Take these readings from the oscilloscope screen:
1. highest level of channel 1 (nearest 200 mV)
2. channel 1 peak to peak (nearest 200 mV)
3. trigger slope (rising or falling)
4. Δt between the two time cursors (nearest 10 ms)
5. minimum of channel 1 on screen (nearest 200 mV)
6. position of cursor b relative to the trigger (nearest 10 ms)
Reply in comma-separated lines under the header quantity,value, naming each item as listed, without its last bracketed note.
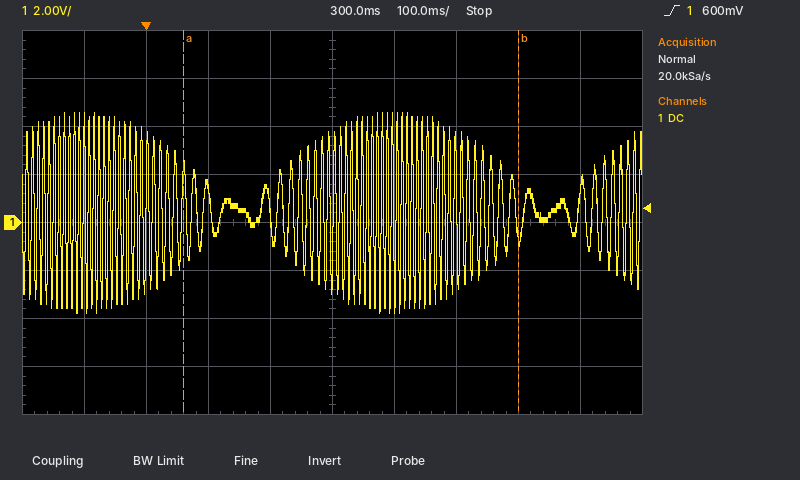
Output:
quantity,value
highest level of channel 1,4.6 V
channel 1 peak to peak,8.4 V
trigger slope,rising
Δt between the two time cursors,540 ms
minimum of channel 1 on screen,-3.8 V
position of cursor b relative to the trigger,+600 ms
